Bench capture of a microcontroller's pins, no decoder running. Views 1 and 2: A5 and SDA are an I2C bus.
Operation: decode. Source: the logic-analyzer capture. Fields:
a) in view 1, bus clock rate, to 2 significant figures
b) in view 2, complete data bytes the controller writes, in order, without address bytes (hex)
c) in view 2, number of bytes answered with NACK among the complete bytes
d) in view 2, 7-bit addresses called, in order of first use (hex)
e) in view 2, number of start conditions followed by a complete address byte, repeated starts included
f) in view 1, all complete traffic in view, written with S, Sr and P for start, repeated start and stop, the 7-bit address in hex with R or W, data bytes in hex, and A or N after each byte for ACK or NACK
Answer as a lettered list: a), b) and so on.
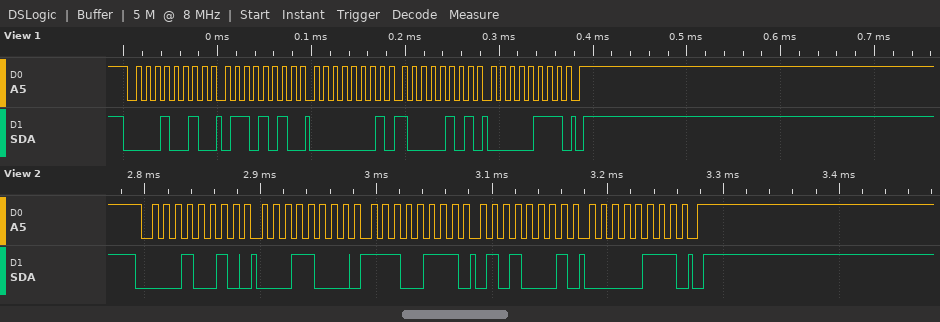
a) 100 kHz
b) 18 E7 51 07
c) 0
d) 0x09
e) 1
f) S 09W A 6A A 01 A 85 A 07 A P
